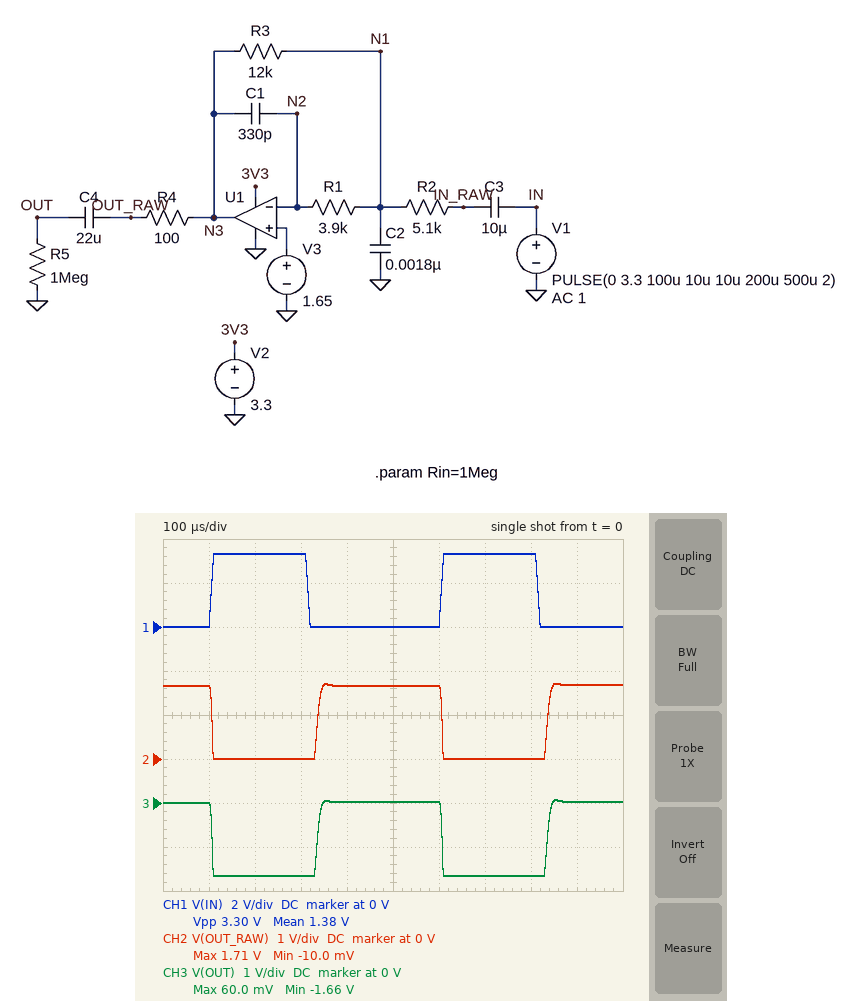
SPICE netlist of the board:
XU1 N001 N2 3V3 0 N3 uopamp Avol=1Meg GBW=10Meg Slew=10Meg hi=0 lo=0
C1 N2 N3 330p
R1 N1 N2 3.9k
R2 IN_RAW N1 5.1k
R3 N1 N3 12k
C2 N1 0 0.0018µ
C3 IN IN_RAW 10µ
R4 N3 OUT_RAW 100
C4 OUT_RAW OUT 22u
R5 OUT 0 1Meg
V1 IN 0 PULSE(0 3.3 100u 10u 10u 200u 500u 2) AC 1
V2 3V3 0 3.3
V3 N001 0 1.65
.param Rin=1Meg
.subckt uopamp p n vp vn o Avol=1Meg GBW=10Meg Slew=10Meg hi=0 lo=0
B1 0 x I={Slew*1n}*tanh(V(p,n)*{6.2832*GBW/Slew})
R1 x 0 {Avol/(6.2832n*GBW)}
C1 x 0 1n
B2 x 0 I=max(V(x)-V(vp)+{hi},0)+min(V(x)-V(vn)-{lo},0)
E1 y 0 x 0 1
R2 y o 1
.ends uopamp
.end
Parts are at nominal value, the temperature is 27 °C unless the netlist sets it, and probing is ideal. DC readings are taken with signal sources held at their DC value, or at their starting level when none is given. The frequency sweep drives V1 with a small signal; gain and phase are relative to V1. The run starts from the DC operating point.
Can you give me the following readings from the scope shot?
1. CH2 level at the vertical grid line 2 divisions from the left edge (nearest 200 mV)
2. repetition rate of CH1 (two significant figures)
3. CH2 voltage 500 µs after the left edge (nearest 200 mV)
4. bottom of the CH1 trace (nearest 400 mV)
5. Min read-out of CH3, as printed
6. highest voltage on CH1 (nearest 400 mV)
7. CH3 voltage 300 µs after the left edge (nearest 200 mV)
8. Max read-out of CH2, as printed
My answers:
0 V
2.0 kHz
1.6 V
0 V
-1.66 V
3.2 V
-1.6 V
1.71 V
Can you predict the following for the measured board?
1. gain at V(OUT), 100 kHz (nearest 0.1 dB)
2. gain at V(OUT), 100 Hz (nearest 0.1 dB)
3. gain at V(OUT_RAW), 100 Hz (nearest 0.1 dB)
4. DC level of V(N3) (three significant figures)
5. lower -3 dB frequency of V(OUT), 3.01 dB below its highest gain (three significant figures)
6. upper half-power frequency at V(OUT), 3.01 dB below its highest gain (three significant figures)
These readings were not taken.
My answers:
-13.7 dB
7.4 dB
7.4 dB
1.65 V
3.12 Hz
26.8 kHz
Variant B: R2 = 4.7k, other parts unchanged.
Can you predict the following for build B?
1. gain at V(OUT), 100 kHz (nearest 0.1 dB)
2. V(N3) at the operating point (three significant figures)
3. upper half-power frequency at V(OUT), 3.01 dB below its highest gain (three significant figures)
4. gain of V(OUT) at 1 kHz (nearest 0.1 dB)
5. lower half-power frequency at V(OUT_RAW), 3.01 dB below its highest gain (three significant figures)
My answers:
-13.0 dB
1.65 V
25.8 kHz
8.1 dB
3.39 Hz
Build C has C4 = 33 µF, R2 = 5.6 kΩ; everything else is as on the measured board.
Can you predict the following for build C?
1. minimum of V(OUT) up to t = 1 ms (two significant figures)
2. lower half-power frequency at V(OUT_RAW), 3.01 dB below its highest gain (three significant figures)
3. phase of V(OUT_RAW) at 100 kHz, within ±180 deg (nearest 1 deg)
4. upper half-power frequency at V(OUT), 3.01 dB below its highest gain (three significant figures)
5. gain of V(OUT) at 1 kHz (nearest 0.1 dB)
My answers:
-1.7 V
2.84 Hz
26 deg
27.9 kHz
6.6 dB
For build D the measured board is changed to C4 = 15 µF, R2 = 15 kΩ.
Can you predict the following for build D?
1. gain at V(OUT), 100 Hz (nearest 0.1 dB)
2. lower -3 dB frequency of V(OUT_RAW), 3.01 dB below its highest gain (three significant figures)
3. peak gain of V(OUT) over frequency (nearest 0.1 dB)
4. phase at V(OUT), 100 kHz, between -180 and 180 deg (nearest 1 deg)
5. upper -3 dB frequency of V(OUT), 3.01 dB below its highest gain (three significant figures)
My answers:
-1.9 dB
1.17 Hz
-1.5 dB
21 deg
33.6 kHz
